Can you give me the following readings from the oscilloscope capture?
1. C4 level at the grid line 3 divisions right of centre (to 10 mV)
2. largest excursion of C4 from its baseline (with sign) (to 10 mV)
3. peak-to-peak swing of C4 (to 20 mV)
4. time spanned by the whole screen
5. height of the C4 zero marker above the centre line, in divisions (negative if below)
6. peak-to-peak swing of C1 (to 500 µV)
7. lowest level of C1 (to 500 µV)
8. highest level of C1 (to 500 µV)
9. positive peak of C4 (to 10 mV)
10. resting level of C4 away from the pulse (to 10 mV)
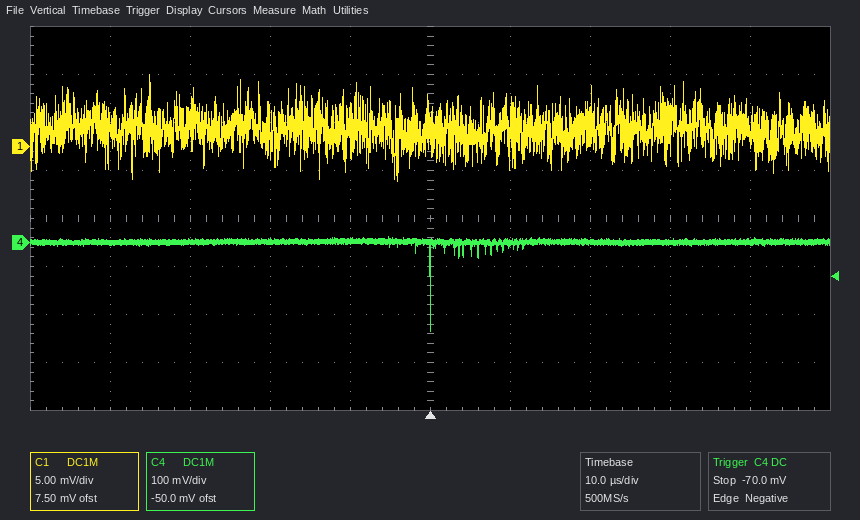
0 mV
-190 mV
200 mV
100 µs
-0.5 div
11.0 mV
-3.5 mV
7.5 mV
10 mV
0 mV
